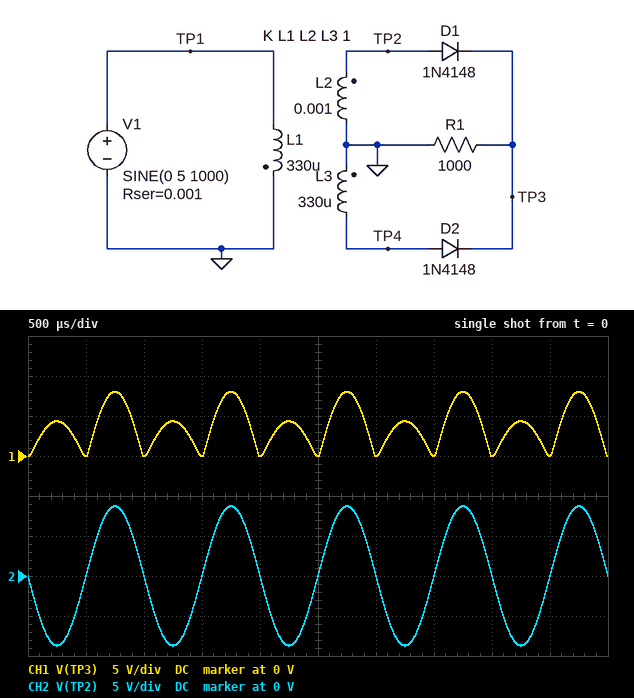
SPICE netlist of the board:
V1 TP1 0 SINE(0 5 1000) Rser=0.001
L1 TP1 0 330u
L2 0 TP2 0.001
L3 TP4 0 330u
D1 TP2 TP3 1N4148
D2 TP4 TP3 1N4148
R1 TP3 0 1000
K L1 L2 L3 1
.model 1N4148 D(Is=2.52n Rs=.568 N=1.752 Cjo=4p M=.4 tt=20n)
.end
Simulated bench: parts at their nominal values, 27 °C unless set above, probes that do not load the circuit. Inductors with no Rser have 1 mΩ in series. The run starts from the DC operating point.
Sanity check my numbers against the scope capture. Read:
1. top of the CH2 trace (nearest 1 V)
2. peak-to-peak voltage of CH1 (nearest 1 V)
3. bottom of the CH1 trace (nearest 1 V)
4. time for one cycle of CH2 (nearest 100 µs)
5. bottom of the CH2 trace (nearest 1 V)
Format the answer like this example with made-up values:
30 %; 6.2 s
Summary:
9 V; 8 V; 0 V; 1.0 ms; -9 V
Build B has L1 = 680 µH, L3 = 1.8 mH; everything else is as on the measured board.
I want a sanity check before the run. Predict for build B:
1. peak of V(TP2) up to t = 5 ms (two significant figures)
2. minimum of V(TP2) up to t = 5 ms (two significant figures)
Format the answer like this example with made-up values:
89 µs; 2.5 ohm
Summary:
6.1 V; -6.1 V
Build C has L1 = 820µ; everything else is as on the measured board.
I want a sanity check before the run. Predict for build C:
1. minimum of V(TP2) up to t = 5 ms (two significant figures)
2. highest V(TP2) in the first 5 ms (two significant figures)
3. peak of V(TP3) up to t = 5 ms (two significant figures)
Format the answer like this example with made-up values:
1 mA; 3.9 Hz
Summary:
-5.5 V; 5.5 V; 4.9 V
